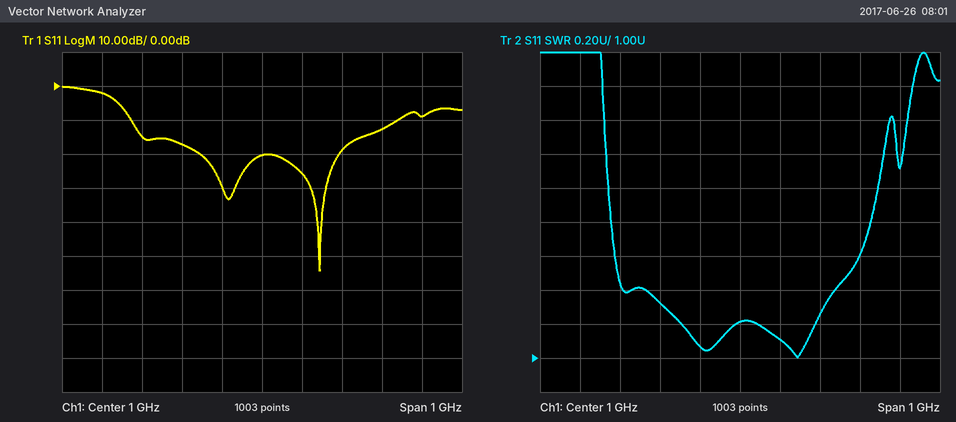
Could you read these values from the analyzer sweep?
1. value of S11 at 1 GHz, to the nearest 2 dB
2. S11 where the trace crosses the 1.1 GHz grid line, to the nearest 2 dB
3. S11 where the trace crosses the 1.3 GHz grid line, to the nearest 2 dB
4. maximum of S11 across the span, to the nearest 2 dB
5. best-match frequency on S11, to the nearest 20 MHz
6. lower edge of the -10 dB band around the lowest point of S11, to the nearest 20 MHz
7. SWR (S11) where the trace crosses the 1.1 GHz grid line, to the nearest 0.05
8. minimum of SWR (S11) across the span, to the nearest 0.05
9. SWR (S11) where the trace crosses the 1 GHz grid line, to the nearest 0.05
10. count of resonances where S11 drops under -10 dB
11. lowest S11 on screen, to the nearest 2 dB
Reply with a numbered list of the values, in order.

1. -20 dB
2. -26 dB
3. -12 dB
4. 0 dB
5. 1.14 GHz
6. 680 MHz
7. 1.10
8. 1.00
9. 1.20
10. 2
11. -54 dB
